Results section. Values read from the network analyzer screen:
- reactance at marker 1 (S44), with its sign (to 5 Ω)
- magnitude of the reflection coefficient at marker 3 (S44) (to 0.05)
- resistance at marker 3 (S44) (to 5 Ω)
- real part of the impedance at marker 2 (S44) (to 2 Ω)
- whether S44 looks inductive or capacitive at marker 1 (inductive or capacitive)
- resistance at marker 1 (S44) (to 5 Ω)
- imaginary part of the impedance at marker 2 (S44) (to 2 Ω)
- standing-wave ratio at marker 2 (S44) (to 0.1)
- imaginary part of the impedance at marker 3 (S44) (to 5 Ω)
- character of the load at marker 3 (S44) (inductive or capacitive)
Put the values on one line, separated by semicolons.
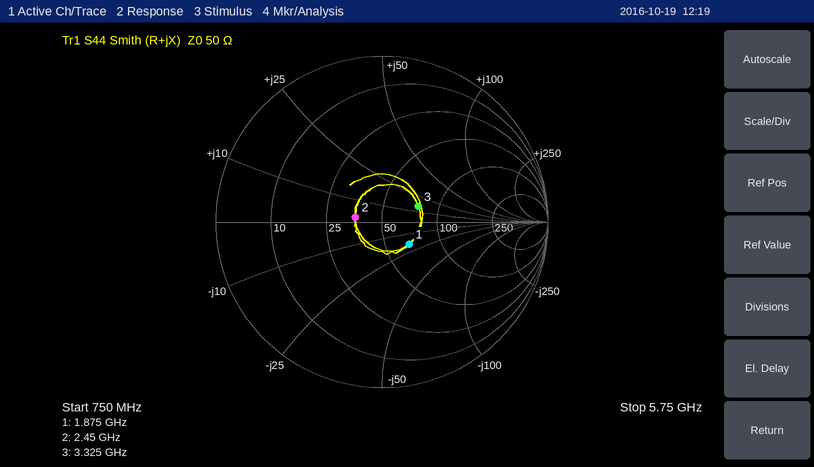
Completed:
-20 Ω; 0.25; 75 Ω; 36 Ω; capacitive; 65 Ω; +2 Ω; 1.4; +15 Ω; inductive
